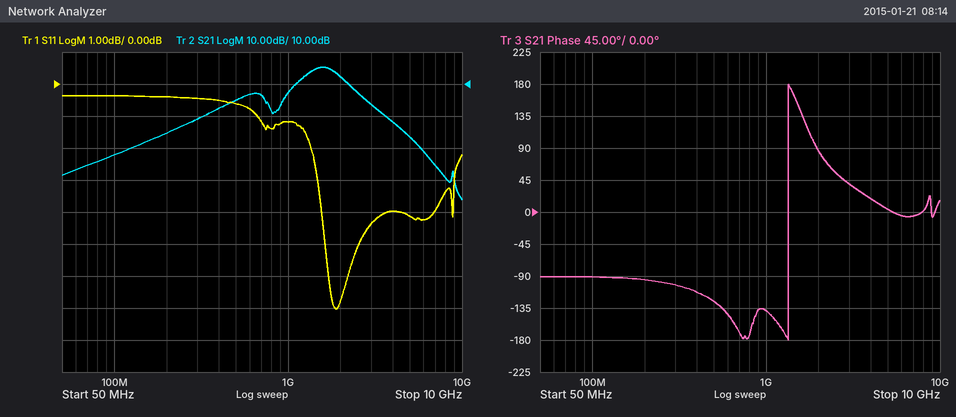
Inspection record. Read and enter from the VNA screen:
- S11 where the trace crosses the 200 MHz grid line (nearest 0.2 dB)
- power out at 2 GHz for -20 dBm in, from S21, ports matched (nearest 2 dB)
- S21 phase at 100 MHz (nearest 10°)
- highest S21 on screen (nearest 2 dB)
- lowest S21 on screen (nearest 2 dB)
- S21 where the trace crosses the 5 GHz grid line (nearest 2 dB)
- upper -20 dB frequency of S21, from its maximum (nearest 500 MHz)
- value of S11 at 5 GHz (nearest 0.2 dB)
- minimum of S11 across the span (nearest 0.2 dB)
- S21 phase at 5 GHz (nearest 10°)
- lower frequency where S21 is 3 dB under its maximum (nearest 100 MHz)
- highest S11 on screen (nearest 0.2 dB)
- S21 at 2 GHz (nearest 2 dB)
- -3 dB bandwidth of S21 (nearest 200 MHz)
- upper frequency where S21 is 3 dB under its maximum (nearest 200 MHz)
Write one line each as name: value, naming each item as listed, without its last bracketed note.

S11 where the trace crosses the 200 MHz grid line: -0.4 dB
power out at 2 GHz for -20 dBm in, from S21, ports matched: -8 dBm
S21 phase at 100 MHz: -90°
highest S21 on screen: 16 dB
lowest S21 on screen: -26 dB
S21 where the trace crosses the 5 GHz grid line: -6 dB
upper -20 dB frequency of S21, from its maximum: 4.5 GHz
value of S11 at 5 GHz: -4.2 dB
minimum of S11 across the span: -7.0 dB
S21 phase at 5 GHz: 0°
lower frequency where S21 is 3 dB under its maximum: 1.2 GHz
highest S11 on screen: -0.4 dB
S21 at 2 GHz: 12 dB
-3 dB bandwidth of S21: 800 MHz
upper frequency where S21 is 3 dB under its maximum: 2.0 GHz
